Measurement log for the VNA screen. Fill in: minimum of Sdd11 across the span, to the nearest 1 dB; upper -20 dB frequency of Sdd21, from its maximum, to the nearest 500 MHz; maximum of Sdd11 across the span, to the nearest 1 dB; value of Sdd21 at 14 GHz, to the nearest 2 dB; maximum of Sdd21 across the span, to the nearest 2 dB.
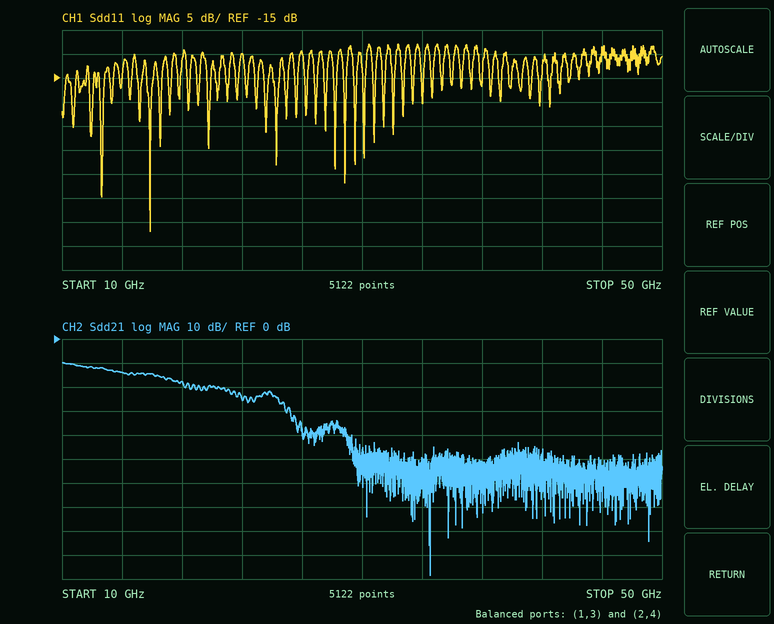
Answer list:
-47 dB
25.0 GHz
-8 dB
-14 dB
-10 dB
